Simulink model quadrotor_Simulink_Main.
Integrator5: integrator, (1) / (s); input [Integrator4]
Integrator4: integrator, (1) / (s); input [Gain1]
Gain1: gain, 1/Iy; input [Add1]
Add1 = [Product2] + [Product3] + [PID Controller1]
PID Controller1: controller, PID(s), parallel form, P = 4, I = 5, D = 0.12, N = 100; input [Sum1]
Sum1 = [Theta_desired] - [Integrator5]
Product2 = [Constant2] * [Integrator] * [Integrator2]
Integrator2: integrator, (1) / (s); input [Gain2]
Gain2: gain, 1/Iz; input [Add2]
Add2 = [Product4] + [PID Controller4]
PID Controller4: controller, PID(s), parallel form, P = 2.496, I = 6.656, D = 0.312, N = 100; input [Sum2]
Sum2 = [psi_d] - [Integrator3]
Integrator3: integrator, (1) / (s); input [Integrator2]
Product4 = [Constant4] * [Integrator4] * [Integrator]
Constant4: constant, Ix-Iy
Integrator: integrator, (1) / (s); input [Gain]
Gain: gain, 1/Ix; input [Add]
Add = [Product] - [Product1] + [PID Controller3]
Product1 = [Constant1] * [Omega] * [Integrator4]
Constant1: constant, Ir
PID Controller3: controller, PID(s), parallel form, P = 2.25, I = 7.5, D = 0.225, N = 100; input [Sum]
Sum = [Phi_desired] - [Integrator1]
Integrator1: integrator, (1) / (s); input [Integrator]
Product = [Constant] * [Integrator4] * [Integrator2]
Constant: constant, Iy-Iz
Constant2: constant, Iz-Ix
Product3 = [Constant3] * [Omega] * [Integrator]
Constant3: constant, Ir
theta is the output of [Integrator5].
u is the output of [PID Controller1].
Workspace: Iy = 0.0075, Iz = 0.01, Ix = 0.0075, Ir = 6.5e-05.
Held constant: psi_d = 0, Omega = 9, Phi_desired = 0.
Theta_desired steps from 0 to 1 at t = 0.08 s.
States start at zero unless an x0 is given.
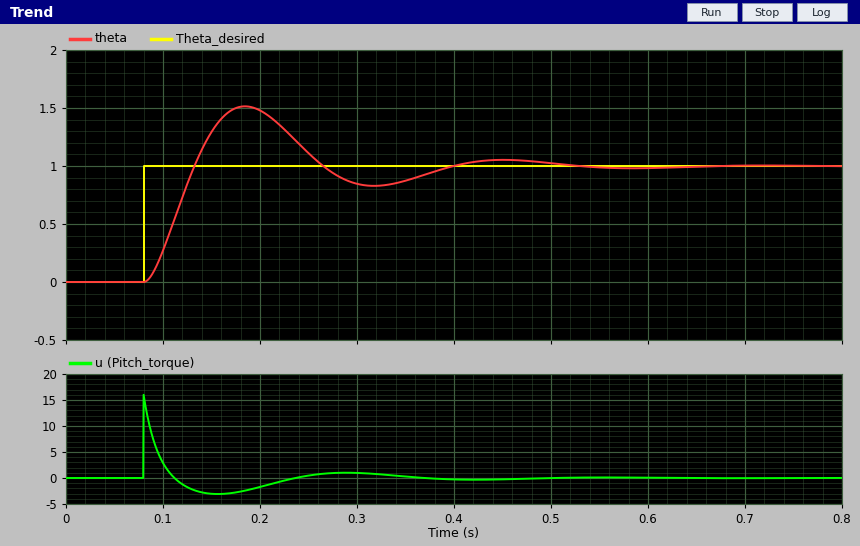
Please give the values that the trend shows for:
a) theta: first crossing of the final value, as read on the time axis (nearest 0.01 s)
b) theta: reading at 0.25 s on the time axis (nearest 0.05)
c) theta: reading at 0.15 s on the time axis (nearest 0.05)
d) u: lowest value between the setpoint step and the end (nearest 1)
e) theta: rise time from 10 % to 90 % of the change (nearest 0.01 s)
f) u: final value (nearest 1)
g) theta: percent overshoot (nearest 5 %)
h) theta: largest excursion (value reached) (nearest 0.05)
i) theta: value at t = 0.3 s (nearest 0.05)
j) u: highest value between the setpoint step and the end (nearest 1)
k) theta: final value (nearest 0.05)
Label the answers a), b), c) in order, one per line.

a) 0.13 s
b) 1.10
c) 1.30
d) -3
e) 0.04 s
f) 0
g) 50 %
h) 1.50
i) 0.85
j) 16
k) 1.00
